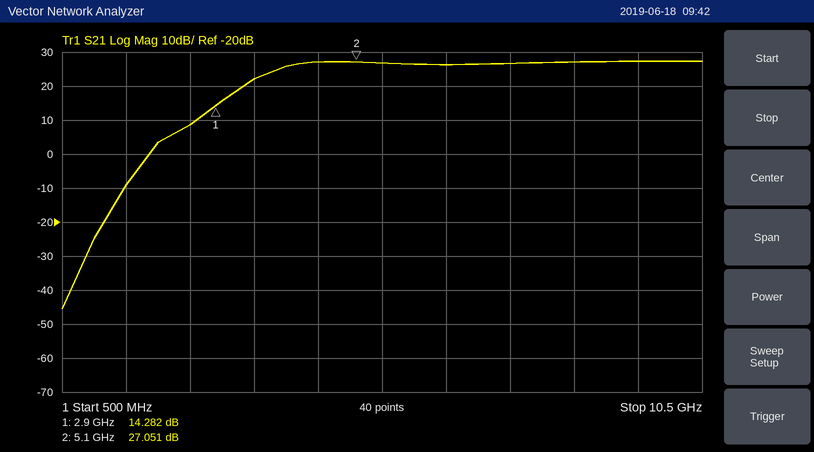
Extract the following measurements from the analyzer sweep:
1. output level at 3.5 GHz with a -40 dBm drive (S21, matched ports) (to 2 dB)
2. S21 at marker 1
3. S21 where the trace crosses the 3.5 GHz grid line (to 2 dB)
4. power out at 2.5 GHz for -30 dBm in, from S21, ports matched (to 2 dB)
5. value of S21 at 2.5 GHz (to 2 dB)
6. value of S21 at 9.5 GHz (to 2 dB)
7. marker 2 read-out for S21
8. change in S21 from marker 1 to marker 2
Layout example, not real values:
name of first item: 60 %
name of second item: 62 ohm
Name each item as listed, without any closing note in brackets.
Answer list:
output level at 3.5 GHz with a -40 dBm drive (S21, matched ports): -18 dBm
S21 at marker 1: 14.282 dB
S21 where the trace crosses the 3.5 GHz grid line: 22 dB
power out at 2.5 GHz for -30 dBm in, from S21, ports matched: -22 dBm
value of S21 at 2.5 GHz: 8 dB
value of S21 at 9.5 GHz: 28 dB
marker 2 read-out for S21: 27.051 dB
change in S21 from marker 1 to marker 2: 12.769 dB
